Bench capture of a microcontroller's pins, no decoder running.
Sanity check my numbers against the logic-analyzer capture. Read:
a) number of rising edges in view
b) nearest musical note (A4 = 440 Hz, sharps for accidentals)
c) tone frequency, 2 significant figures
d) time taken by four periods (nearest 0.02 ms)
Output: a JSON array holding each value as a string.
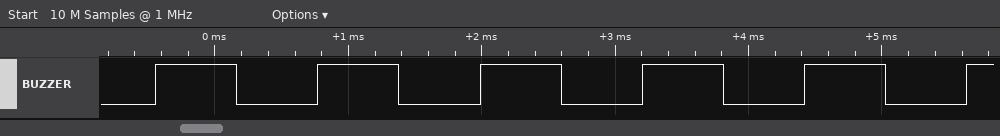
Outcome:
["6", "G#5", "820 Hz", "4.86 ms"]
